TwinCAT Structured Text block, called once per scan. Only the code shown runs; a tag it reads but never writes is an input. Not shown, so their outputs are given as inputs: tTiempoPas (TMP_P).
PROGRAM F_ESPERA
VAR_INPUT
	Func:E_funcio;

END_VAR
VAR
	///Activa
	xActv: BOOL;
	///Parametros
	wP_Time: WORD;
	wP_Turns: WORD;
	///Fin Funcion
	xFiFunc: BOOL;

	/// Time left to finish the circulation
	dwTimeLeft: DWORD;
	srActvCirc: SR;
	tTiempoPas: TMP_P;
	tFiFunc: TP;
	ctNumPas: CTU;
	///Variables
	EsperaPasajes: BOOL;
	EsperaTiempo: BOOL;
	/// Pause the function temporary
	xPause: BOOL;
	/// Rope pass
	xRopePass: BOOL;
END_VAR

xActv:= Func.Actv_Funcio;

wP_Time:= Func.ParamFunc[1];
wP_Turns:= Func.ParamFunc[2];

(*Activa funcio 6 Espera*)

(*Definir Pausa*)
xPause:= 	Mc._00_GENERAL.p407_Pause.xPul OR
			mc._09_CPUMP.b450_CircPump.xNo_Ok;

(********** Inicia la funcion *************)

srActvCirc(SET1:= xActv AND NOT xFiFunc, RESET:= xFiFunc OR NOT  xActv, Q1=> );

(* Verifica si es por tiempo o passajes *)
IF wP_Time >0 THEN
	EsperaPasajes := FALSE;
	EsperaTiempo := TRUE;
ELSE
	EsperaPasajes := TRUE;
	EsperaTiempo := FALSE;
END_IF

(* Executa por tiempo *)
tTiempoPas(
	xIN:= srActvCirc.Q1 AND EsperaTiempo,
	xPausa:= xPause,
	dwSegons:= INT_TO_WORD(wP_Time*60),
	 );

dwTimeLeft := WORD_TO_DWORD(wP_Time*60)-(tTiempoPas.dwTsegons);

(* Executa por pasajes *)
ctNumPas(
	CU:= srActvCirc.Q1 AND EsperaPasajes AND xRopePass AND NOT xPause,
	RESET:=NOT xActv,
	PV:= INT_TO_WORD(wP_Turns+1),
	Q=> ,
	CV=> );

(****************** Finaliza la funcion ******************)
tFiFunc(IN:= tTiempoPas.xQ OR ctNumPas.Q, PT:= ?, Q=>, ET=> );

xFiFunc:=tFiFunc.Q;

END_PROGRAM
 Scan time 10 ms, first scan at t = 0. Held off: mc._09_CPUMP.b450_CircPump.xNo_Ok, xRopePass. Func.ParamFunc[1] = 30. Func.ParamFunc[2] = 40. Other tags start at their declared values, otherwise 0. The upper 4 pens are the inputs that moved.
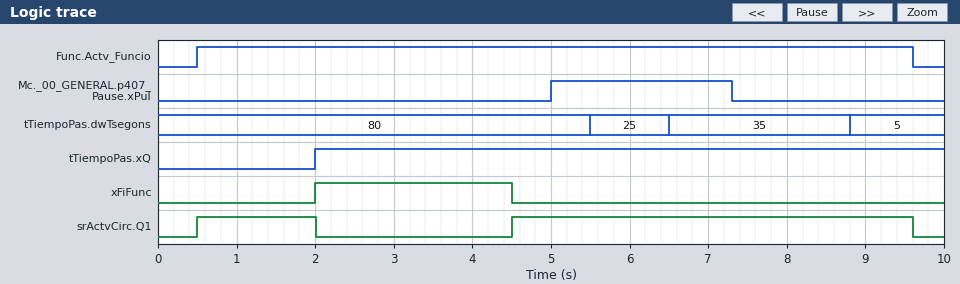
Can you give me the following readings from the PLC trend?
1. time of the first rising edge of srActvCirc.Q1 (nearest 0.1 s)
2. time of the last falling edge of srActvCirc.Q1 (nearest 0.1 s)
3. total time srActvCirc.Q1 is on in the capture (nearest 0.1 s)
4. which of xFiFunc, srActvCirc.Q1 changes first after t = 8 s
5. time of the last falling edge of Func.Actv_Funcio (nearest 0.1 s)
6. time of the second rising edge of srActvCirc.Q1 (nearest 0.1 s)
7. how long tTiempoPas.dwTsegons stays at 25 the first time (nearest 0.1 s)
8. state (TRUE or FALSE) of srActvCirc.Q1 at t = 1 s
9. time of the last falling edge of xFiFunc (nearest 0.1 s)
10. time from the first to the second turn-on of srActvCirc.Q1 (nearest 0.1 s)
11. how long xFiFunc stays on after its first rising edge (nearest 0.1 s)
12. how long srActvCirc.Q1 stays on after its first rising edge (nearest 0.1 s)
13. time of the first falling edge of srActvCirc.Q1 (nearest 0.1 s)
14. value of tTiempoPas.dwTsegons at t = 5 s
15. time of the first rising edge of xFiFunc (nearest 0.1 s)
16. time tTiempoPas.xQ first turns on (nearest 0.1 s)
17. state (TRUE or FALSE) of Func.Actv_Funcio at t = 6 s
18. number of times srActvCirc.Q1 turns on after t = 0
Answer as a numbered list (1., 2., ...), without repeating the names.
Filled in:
1. 0.5 s
2. 9.6 s
3. 6.6 s
4. srActvCirc.Q1
5. 9.6 s
6. 4.5 s
7. 1.0 s
8. TRUE
9. 4.5 s
10. 4.0 s
11. 2.5 s
12. 1.5 s
13. 2.0 s
14. 80
15. 2.0 s
16. 2.0 s
17. TRUE
18. 2
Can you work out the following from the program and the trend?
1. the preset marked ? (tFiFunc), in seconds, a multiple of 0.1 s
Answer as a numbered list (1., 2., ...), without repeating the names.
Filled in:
1. 2.5 s
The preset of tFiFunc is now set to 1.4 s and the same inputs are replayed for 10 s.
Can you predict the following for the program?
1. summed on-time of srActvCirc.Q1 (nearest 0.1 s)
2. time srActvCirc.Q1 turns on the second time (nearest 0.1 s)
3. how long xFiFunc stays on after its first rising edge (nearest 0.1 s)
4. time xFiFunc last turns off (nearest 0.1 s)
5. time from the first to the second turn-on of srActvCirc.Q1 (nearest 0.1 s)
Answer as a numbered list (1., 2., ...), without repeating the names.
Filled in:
1. 7.7 s
2. 3.4 s
3. 1.4 s
4. 3.4 s
5. 2.9 s
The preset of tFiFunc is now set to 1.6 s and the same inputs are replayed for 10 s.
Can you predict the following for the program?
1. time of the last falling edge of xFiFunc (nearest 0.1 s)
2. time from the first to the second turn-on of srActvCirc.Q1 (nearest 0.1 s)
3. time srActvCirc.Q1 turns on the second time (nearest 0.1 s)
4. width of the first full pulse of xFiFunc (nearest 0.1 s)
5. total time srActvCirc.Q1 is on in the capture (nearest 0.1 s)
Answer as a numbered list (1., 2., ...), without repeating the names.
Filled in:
1. 3.6 s
2. 3.1 s
3. 3.6 s
4. 1.6 s
5. 7.5 s
